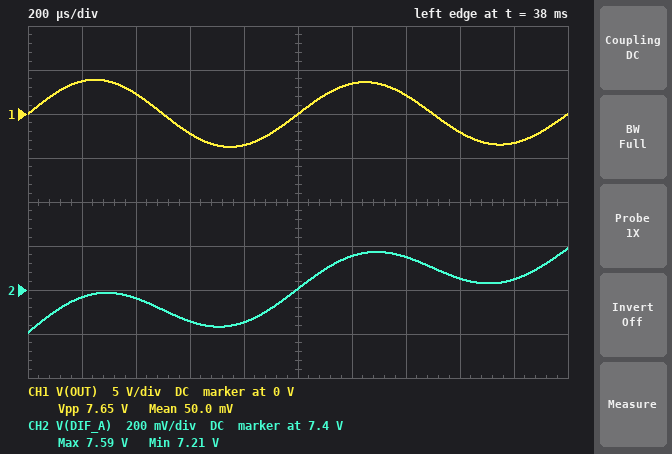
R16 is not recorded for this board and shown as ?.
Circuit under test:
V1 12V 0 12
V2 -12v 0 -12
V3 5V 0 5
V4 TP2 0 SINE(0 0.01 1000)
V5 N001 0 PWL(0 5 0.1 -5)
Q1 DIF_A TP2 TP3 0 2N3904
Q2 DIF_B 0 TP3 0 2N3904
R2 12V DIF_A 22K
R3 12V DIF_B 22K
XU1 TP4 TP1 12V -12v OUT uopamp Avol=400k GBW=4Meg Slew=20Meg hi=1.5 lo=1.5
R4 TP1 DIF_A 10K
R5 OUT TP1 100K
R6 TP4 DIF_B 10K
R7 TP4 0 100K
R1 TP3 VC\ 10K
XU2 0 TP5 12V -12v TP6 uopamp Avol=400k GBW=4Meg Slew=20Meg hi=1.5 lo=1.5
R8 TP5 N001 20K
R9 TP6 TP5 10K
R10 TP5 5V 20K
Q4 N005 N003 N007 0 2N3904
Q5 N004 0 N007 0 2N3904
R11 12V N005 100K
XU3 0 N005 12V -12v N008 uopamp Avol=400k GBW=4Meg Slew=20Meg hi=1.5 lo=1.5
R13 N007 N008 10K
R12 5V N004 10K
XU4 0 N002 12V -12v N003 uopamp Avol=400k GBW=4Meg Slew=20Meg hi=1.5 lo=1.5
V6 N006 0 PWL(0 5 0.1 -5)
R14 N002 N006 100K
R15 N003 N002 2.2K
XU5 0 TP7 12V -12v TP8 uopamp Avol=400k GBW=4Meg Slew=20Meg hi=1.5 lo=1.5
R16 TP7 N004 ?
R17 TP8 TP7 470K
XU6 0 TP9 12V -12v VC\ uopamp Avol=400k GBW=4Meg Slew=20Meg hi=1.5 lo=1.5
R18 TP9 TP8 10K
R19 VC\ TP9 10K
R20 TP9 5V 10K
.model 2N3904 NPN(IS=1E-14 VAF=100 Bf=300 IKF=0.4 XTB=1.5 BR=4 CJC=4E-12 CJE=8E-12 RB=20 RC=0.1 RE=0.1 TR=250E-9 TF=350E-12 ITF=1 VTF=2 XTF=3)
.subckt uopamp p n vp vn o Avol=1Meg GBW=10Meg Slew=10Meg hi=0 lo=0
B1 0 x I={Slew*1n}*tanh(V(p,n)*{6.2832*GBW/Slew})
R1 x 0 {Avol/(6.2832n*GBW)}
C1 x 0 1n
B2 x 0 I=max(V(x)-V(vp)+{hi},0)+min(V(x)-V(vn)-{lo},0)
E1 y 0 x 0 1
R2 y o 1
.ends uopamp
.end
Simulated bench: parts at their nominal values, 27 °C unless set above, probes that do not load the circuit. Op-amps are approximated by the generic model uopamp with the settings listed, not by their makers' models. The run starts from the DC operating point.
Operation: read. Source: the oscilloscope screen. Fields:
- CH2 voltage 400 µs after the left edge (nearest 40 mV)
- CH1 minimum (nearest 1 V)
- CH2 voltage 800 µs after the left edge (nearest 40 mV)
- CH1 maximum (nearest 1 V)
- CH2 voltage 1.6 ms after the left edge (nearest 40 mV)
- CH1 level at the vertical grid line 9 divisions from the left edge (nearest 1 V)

7.36 V
-4 V
7.24 V
4 V
7.44 V
-3 V
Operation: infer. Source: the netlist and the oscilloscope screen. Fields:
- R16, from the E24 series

560 kΩ
